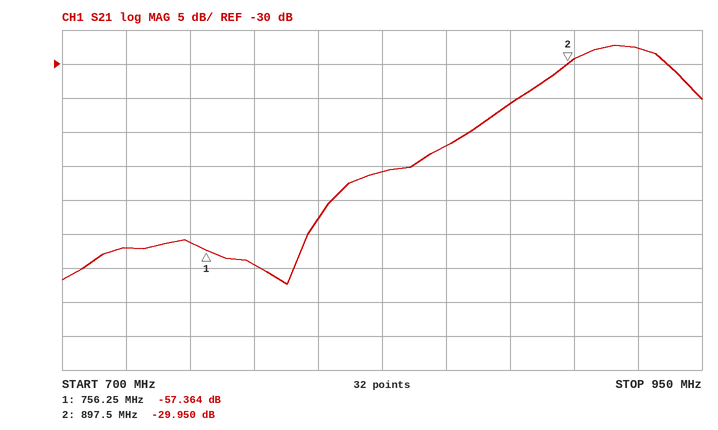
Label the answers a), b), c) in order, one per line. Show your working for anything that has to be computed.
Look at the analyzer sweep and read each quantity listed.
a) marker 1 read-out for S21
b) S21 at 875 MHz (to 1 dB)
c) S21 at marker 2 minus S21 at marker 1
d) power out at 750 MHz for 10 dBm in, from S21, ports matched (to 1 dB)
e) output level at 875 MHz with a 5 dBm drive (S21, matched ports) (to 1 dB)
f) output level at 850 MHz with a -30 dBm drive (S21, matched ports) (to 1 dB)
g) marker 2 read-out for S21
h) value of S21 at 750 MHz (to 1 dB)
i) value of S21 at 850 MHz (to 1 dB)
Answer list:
a) -57.364 dB
b) -36 dB
c) -29.95 − (-57.364) = 27.414 dB
d) 10 dBm + (-56 dB) = -46 dBm
e) 5 dBm + (-36 dB) = -31 dBm
f) -30 dBm + (-42 dB) = -72 dBm
g) -29.950 dB
h) -56 dB
i) -42 dB
